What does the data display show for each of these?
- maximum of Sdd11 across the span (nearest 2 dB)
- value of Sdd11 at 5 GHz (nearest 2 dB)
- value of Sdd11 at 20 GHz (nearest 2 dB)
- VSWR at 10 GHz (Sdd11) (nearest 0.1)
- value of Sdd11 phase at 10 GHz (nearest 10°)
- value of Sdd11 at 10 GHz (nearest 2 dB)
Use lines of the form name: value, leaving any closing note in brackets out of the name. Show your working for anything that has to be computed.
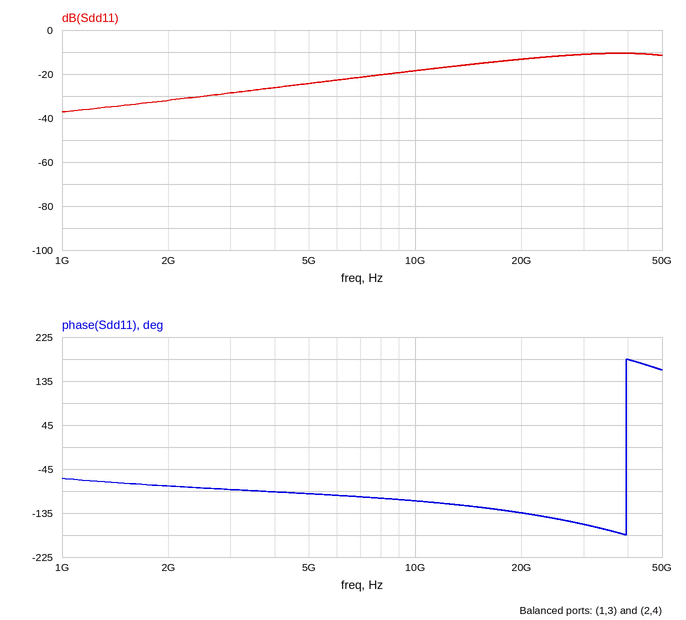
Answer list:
maximum of Sdd11 across the span: -10 dB
value of Sdd11 at 5 GHz: -24 dB
value of Sdd11 at 20 GHz: -14 dB
VSWR at 10 GHz (Sdd11): |Γ| = 10^(-18/20) = 0.1259; VSWR = (1 + 0.1259)/(1 − 0.1259) ≈ 1.3
value of Sdd11 phase at 10 GHz: -110°
value of Sdd11 at 10 GHz: -18 dB
